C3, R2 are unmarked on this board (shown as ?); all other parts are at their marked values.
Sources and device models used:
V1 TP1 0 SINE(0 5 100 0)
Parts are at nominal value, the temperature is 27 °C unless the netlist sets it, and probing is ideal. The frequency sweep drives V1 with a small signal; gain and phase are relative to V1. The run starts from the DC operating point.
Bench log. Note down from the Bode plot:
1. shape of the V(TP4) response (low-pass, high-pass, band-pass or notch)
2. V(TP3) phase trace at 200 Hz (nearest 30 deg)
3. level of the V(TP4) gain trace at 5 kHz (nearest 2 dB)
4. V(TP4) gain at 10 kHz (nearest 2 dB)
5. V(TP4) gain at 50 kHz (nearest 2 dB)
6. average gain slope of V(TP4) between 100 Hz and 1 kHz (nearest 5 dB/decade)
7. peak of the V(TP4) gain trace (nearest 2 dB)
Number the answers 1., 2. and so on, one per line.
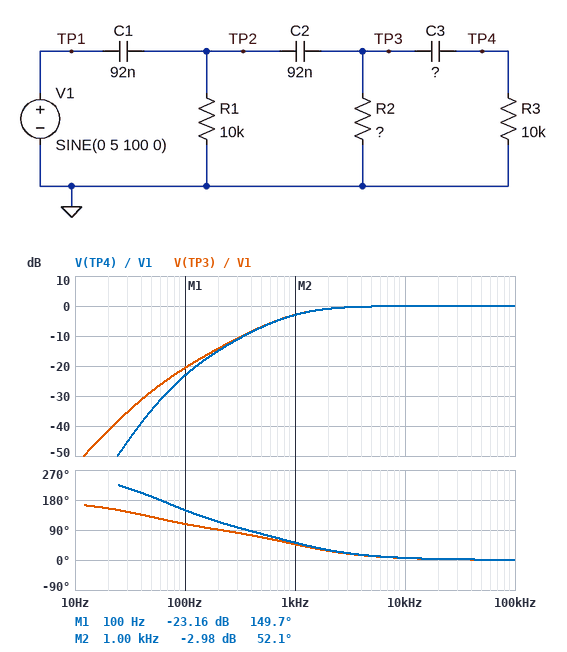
1. high-pass
2. 90 deg
3. 0 dB
4. 0 dB
5. 0 dB
6. 20 dB/decade
7. 0 dB
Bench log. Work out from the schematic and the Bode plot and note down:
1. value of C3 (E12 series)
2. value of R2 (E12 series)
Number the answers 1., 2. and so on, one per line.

1. 180 nF
2. 6.8 kΩ
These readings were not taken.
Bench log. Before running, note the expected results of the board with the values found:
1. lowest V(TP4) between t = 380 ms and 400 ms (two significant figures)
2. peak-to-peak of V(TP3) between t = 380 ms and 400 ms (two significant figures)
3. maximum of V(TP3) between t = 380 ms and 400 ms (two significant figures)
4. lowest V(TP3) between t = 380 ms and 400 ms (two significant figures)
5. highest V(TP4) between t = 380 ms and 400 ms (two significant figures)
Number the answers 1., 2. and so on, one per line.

1. -350 mV
2. 930 mV
3. 460 mV
4. -460 mV
5. 350 mV
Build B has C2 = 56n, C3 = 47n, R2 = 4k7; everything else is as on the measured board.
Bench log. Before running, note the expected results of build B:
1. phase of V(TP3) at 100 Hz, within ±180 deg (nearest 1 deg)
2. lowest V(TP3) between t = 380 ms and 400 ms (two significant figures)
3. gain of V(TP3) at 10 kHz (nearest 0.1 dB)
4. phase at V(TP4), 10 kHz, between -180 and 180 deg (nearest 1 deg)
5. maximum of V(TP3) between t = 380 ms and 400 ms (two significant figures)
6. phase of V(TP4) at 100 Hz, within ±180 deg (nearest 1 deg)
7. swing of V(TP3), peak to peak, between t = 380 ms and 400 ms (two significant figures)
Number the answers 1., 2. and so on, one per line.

1. 123 deg
2. -320 mV
3. -0.1 dB
4. 11 deg
5. 320 mV
6. -163 deg
7. 640 mV
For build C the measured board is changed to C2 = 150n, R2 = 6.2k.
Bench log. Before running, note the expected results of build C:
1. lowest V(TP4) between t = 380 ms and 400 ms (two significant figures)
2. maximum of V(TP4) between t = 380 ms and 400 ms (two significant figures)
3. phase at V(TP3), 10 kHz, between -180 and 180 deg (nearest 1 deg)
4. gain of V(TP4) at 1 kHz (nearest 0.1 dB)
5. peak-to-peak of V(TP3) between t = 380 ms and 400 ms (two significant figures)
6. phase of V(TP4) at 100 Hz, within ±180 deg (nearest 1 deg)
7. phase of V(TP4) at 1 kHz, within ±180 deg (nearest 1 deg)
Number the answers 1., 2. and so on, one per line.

1. -420 mV
2. 420 mV
3. 5 deg
4. -2.5 dB
5. 1.1 V
6. 142 deg
7. 48 deg
